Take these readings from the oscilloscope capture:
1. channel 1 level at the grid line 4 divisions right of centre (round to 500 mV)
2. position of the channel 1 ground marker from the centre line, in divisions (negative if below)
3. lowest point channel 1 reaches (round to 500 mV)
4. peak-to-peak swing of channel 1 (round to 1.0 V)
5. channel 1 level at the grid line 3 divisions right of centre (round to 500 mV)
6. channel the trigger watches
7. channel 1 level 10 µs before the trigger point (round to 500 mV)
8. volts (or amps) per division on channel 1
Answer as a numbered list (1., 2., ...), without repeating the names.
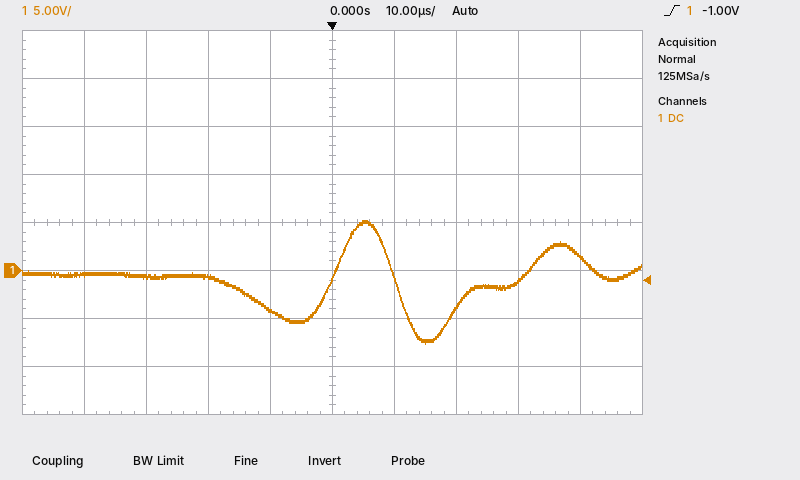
1. 1.5 V
2. -1.0 div
3. -7.5 V
4. 13.0 V
5. -1.0 V
6. channel 1
7. -4.0 V
8. 5 V
